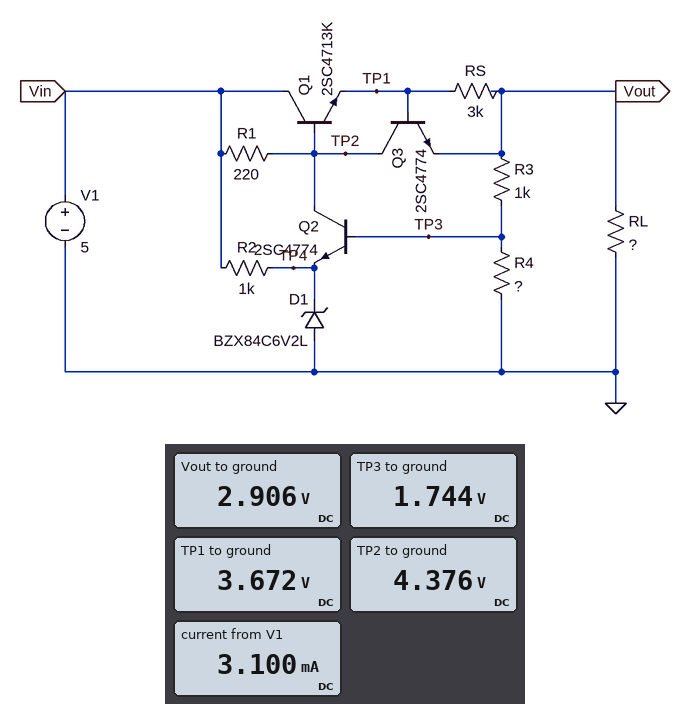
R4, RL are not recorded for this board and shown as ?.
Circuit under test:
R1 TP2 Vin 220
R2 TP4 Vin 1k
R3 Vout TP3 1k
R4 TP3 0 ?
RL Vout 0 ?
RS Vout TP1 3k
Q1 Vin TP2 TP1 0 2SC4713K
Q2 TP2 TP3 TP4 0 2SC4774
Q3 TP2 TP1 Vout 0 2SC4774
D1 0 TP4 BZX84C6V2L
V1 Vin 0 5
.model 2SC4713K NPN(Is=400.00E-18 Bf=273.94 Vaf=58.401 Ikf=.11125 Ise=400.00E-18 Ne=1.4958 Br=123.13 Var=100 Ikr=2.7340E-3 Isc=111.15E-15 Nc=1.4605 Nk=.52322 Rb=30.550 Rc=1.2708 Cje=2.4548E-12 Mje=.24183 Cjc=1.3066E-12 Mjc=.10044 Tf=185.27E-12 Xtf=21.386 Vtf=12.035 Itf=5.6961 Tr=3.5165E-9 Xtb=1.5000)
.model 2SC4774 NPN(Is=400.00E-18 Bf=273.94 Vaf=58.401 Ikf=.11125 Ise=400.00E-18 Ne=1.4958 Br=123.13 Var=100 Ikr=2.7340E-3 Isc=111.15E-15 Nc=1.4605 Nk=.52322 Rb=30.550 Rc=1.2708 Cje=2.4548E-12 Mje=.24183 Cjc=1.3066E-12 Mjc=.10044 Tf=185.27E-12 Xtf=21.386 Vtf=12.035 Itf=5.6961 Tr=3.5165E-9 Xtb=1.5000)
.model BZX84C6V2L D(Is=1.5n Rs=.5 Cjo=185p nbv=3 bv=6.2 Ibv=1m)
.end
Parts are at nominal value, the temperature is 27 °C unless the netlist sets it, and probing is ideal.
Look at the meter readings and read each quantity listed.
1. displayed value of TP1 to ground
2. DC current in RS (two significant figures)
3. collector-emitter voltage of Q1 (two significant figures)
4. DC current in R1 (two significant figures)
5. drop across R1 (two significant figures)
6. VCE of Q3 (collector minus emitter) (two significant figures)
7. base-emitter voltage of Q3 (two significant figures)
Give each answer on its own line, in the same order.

3.672 V
260 µA
1.3 V
2.8 mA
620 mV
1.5 V
770 mV
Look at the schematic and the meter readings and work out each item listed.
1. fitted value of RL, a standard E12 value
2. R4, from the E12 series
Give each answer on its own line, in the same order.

1.5 kΩ
1.5 kΩ
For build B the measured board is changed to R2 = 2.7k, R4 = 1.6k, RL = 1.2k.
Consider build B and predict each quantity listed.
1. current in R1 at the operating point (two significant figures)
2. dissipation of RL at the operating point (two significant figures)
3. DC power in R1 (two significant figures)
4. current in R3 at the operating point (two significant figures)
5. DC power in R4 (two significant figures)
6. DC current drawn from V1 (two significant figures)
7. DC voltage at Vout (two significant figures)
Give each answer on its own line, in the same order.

3.2 mA
6.7 mW
2.2 mW
1.1 mA
1.9 mW
3.4 mA
2.8 V
